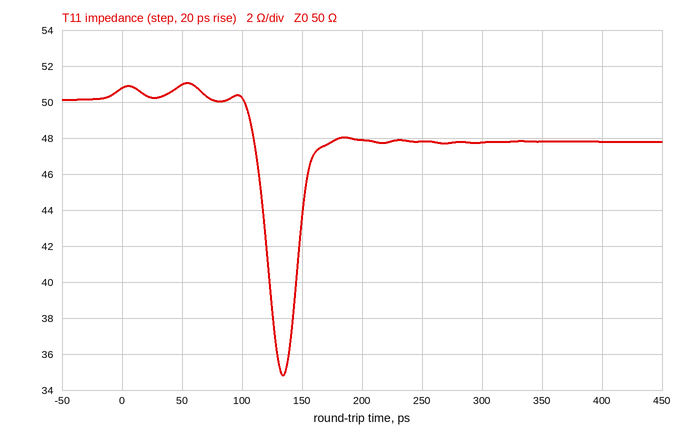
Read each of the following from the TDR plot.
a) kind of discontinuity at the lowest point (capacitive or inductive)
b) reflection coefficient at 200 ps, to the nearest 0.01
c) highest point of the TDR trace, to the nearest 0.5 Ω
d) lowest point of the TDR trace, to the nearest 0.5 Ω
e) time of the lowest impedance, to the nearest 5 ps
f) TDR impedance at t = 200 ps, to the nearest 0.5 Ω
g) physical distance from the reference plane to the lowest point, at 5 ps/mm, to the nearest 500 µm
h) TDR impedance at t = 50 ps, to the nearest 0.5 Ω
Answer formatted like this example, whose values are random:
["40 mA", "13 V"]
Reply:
["capacitive", "-0.02", "51.0 Ω", "35.0 Ω", "135 ps", "48.0 Ω", "13.5 mm", "51.0 Ω"]
